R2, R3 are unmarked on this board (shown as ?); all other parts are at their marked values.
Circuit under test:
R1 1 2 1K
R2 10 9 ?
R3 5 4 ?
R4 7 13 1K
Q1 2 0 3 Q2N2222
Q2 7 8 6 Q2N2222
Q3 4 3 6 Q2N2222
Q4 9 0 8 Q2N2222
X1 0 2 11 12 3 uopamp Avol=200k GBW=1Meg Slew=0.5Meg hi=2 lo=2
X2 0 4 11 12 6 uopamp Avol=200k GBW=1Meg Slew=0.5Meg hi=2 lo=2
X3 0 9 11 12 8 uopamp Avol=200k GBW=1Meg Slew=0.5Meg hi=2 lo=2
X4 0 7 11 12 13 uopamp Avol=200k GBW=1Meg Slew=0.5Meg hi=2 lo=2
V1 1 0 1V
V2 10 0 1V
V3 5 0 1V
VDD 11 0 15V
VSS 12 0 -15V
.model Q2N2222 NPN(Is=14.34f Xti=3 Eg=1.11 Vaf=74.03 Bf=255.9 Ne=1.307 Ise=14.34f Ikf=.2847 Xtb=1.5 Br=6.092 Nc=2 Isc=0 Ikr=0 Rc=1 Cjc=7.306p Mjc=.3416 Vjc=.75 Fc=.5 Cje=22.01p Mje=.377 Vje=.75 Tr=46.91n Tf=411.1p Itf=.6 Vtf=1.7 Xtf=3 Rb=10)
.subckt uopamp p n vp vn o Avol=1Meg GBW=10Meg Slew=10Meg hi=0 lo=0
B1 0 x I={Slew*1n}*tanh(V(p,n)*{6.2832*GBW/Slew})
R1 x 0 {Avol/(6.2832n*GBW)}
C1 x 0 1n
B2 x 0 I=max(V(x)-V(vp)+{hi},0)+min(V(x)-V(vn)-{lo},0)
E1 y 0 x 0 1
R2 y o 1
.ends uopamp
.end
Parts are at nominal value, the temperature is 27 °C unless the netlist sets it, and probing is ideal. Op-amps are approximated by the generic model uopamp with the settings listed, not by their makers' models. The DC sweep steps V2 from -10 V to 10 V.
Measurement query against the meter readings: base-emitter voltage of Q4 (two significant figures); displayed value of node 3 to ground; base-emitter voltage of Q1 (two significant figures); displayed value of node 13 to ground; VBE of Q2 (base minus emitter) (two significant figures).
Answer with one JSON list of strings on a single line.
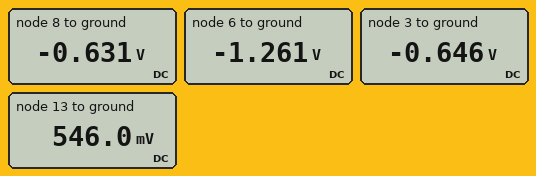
["630 mV", "-0.646 V", "650 mV", "546.0 mV", "630 mV"]
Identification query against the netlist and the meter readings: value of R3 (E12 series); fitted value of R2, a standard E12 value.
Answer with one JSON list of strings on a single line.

["3.3 kΩ", "1.8 kΩ"]
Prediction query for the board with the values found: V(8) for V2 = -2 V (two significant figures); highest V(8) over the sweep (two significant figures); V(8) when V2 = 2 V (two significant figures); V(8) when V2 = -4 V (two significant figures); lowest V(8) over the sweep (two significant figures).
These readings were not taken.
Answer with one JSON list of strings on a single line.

["12 V", "12 V", "-650 mV", "12 V", "-690 mV"]
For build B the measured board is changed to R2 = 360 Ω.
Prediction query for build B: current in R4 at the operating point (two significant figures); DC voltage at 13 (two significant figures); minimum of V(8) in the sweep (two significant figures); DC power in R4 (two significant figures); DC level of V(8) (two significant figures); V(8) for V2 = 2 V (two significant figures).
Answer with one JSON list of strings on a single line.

["110 µA", "110 mV", "-740 mV", "12 µW", "-670 mV", "-690 mV"]
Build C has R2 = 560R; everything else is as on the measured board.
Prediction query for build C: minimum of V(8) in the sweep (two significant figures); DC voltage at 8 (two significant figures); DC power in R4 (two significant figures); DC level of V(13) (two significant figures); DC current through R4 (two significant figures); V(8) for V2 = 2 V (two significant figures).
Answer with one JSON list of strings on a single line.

["-720 mV", "-660 mV", "29 µW", "170 mV", "170 µA", "-680 mV"]
